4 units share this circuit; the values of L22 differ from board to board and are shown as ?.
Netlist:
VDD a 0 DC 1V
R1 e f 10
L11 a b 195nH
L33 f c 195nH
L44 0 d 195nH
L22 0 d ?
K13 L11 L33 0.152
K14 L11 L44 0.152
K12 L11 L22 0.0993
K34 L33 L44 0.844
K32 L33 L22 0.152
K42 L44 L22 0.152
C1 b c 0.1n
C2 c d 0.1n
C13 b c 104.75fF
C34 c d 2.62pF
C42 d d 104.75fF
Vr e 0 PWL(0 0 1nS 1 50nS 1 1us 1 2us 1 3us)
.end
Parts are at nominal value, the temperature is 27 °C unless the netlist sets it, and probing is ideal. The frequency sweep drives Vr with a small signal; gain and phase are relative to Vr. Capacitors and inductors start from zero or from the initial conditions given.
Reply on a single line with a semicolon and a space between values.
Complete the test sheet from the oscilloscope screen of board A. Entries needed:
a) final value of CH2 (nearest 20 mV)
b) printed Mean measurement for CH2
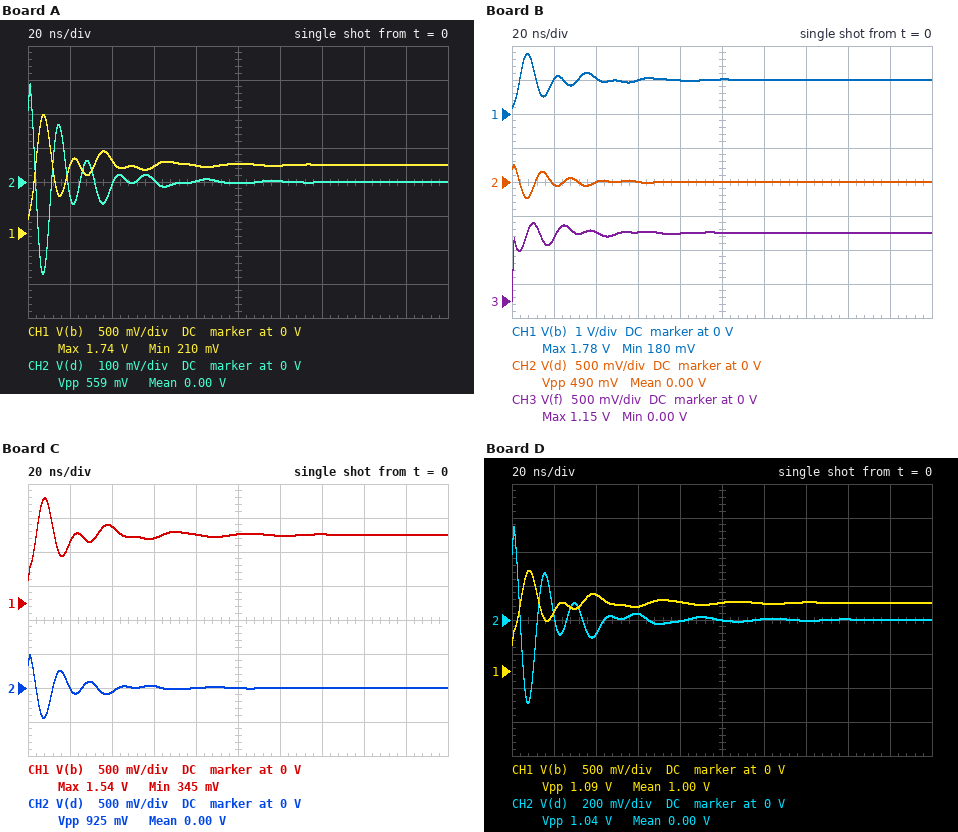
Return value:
0 V; 0.00 V
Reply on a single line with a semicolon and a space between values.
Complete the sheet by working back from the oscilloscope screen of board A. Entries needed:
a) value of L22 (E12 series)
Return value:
82 nH
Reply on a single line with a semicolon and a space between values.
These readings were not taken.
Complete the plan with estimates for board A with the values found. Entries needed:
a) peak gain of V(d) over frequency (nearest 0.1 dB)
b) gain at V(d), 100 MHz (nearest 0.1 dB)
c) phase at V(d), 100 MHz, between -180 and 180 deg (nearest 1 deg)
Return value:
0.1 dB; -9.3 dB; 27 deg
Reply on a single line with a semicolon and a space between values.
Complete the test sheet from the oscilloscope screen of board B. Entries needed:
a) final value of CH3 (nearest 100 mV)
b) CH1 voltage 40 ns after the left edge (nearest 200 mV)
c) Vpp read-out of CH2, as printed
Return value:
1.0 V; 1.0 V; 490 mV
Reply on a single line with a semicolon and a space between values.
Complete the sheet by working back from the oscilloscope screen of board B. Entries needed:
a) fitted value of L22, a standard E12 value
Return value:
68 nH
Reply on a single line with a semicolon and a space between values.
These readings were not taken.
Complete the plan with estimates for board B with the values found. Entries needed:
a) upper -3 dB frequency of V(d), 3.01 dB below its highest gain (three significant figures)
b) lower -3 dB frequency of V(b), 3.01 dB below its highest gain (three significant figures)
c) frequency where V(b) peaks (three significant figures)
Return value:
81.0 MHz; 28.4 MHz; 32.2 MHz
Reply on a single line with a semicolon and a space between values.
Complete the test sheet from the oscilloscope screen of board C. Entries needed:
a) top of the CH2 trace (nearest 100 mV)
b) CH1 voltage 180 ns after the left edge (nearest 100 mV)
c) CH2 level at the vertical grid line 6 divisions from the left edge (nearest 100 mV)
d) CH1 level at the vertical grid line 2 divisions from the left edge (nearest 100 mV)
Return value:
500 mV; 1.0 V; 0 V; 1.1 V
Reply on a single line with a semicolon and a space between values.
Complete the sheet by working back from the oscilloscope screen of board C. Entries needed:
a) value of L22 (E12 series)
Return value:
220 nH
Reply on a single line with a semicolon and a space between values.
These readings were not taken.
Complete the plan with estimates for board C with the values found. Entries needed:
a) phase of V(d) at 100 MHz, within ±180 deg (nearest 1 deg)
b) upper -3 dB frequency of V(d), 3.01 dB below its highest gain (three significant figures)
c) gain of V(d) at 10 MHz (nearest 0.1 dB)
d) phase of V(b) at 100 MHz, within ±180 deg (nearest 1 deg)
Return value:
26 deg; 77.8 MHz; -31.1 dB; -154 deg
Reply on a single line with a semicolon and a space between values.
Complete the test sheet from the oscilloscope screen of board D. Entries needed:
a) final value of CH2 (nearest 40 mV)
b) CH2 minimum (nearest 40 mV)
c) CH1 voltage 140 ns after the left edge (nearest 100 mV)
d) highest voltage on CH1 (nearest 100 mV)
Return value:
0 V; -480 mV; 1.0 V; 1.5 V
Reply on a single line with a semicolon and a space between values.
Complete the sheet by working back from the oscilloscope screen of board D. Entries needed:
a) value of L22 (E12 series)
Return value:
330 nH
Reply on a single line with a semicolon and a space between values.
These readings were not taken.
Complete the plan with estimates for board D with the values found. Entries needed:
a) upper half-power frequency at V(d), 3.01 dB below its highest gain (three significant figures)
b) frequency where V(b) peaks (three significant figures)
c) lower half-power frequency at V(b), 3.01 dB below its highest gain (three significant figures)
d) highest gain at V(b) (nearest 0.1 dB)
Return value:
76.9 MHz; 30.0 MHz; 26.9 MHz; 8.7 dB
